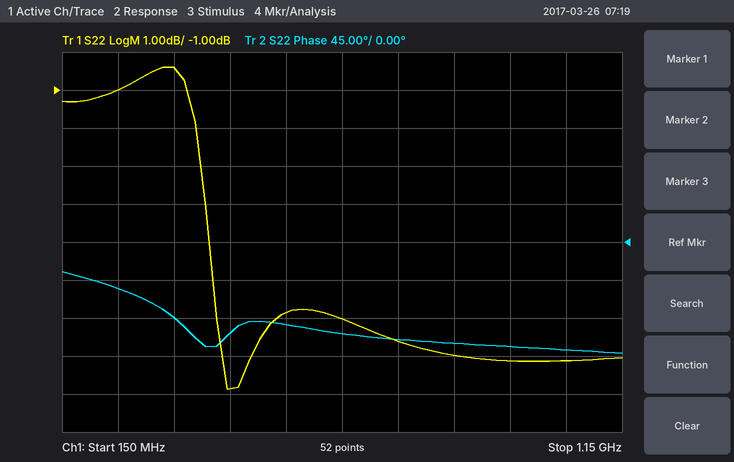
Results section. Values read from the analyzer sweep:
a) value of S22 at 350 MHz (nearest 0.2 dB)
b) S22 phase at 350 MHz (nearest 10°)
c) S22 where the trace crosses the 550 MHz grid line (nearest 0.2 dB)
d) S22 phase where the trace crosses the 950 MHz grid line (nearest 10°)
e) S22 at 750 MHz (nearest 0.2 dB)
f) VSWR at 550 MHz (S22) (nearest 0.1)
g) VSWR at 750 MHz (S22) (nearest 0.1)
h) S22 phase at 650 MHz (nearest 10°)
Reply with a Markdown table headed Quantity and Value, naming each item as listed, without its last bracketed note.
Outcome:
| Quantity | Value |
|---|---|
| value of S22 at 350 MHz | -0.4 dB |
| S22 phase at 350 MHz | -90° |
| S22 where the trace crosses the 550 MHz grid line | -6.8 dB |
| S22 phase where the trace crosses the 950 MHz grid line | -120° |
| S22 at 750 MHz | -7.6 dB |
| VSWR at 550 MHz (S22) | 2.7 |
| VSWR at 750 MHz (S22) | 2.4 |
| S22 phase at 650 MHz | -110° |
